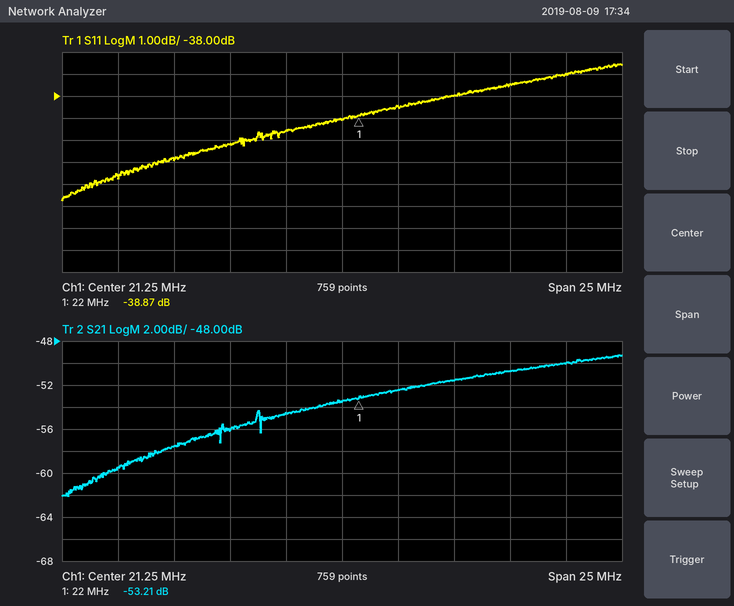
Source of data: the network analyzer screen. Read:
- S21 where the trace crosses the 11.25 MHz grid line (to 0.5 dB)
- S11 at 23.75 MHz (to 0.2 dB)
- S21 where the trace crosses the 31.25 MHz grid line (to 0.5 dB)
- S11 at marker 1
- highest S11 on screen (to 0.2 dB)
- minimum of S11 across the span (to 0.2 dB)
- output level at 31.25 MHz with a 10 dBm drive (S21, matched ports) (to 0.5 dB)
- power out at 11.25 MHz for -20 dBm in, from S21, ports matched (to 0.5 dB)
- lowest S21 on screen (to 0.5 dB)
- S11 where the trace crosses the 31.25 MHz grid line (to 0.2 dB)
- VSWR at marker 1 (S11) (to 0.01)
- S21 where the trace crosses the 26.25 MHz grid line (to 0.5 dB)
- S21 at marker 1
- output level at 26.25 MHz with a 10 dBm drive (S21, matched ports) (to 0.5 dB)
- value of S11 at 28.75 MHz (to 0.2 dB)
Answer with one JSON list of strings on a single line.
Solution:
["-59.5 dB", "-38.4 dB", "-50.0 dB", "-38.87 dB", "-36.6 dB", "-42.8 dB", "-40.0 dBm", "-79.5 dBm", "-62.0 dB", "-37.0 dB", "1.02", "-51.5 dB", "-53.21 dB", "-41.5 dBm", "-37.4 dB"]
